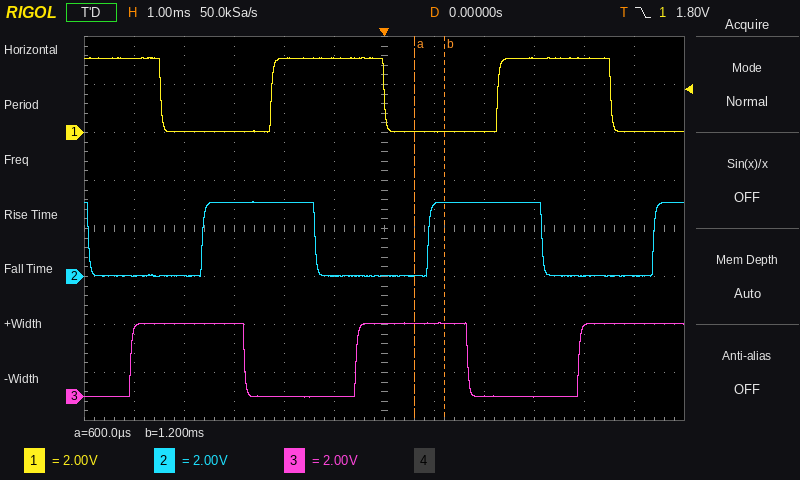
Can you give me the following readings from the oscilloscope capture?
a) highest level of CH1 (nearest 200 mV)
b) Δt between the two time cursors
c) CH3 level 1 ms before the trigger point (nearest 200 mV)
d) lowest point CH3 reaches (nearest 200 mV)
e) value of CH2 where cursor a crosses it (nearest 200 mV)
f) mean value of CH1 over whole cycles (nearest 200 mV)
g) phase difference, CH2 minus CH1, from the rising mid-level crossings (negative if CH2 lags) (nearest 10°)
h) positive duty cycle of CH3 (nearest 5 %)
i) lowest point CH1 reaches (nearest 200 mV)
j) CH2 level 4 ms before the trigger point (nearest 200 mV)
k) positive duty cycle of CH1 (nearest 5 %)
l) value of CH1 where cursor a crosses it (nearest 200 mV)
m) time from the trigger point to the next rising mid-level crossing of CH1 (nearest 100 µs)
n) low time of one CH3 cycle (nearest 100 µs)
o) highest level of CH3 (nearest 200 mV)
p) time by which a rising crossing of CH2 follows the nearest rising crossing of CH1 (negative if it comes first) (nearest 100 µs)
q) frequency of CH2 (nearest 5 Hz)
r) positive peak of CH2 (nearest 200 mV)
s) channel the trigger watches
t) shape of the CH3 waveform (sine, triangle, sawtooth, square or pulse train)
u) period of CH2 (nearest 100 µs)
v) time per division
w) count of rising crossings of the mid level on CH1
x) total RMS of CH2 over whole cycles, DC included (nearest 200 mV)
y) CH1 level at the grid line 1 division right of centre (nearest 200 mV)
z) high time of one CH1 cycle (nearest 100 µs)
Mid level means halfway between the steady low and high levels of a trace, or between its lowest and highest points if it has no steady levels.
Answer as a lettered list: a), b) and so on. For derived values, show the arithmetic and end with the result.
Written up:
a) 3.2 V
b) 1.2 ms − (600 µs) = 600 µs
c) 0.0 V
d) 0.0 V
e) 0.0 V
f) 0.0 V + 0.5 × (3.2 V − (0.0 V)) ≈ 1.6 V
g) −360° × (-1.4 ms) / 4.5 ms ≈ +112°, so +110° to the nearest 10°
h) 50 %
i) 0.0 V
j) 0.0 V
k) 2.3 ms / 4.5 ms ≈ 51.1 %, so 50 % to the nearest 5 %
l) 0.0 V
m) 2.3 ms
n) 2.2 ms
o) 3.0 V
p) -1.4 ms
q) 1 / 4.5 ms ≈ 222 Hz, so 220 Hz to the nearest 5 Hz
r) 3.2 V
s) CH1
t) square
u) 4.5 ms
v) 1 ms
w) 2
x) √(0.5 × (3.2 V)² + 0.5 × (0.0 V)²) ≈ 2.26 V, so 2.2 V to the nearest 200 mV
y) 0.0 V
z) 2.3 ms
